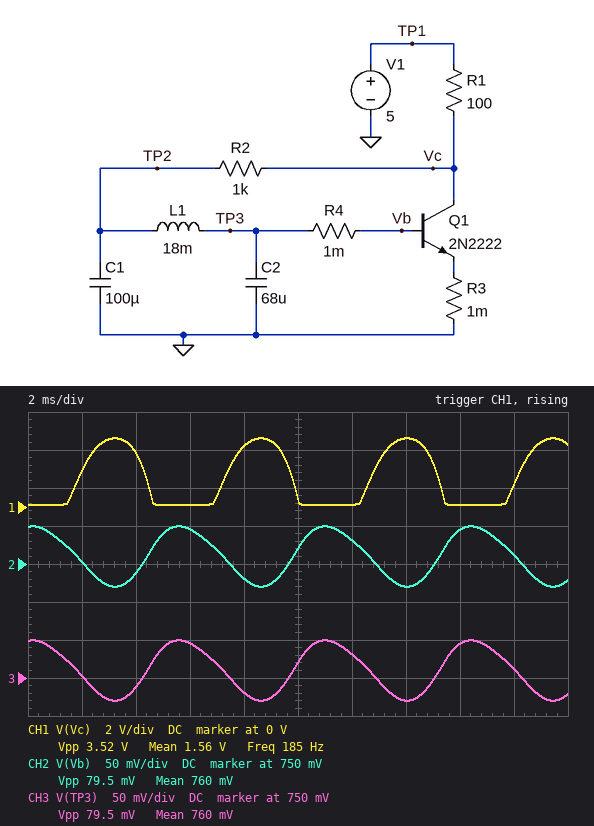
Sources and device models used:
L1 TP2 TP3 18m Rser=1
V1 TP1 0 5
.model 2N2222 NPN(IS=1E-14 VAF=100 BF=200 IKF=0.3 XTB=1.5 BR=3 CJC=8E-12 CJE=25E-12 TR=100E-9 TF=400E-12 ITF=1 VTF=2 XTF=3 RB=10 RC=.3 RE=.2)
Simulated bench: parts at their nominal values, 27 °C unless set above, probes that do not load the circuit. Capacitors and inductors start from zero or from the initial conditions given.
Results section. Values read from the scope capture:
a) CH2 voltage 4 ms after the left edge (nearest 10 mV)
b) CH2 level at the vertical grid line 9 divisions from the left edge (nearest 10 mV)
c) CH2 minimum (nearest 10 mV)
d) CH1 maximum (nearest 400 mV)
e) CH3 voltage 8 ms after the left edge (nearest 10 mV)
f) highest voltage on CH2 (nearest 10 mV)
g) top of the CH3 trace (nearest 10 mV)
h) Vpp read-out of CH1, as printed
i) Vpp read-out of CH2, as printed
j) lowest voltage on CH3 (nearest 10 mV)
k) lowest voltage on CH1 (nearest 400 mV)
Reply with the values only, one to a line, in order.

740 mV
760 mV
720 mV
3.6 V
730 mV
800 mV
800 mV
3.52 V
79.5 mV
720 mV
0 V
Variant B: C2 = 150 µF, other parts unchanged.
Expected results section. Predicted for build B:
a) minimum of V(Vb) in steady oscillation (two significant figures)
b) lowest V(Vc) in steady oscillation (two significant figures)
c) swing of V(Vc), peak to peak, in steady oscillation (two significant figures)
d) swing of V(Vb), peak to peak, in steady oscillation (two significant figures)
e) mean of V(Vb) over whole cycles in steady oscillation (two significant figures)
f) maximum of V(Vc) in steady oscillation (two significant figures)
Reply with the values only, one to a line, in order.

680 mV
73 mV
4.3 V
150 mV
750 mV
4.4 V
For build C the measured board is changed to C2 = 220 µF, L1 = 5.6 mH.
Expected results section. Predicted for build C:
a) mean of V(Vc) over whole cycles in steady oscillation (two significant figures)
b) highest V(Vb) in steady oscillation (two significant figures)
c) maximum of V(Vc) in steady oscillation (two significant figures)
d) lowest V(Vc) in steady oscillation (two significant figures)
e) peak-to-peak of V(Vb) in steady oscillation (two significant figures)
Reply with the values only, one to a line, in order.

1.1 V
780 mV
2.5 V
110 mV
37 mV
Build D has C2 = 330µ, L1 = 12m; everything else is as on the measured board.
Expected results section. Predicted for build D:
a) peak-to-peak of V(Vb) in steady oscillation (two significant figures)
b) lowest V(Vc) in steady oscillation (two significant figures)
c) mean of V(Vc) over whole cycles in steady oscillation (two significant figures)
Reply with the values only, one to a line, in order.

82 mV
85 mV
1.6 V
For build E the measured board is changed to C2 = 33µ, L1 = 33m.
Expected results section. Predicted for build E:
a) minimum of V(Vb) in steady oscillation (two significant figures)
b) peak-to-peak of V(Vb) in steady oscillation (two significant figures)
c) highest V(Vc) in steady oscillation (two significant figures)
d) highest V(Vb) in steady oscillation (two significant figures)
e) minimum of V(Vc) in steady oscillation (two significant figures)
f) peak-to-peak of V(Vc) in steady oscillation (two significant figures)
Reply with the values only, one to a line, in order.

730 mV
52 mV
3.0 V
790 mV
100 mV
2.9 V
